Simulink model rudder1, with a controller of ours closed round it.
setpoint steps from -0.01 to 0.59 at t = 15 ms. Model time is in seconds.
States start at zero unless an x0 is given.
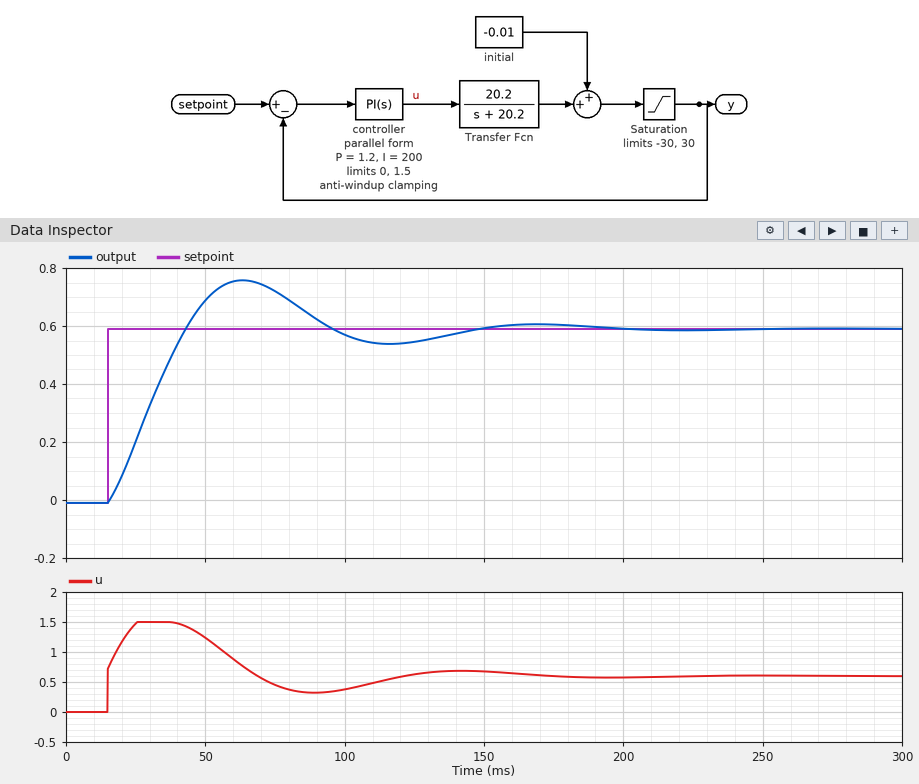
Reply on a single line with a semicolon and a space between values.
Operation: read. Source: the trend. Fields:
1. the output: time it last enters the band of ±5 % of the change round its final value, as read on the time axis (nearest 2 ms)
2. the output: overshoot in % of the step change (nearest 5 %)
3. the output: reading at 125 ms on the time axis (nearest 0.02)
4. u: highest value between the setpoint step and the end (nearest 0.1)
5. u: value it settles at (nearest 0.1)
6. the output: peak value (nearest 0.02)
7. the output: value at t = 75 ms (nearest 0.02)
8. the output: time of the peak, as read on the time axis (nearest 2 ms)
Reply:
134 ms; 30 %; 0.54; 1.5; 0.6; 0.76; 0.72; 64 ms
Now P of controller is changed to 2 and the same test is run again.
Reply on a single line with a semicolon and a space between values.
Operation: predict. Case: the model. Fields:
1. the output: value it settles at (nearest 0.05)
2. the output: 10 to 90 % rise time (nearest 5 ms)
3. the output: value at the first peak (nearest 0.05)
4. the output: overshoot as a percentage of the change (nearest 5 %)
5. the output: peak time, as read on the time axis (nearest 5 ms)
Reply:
0.60; 20 ms; 0.70; 20 %; 60 ms
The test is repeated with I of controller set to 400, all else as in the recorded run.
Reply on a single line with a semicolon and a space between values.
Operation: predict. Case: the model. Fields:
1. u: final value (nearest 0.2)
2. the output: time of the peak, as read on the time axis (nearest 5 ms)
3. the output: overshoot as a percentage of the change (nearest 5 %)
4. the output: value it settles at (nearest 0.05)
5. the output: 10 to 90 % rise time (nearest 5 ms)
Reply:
0.6; 55 ms; 25 %; 0.60; 20 ms
